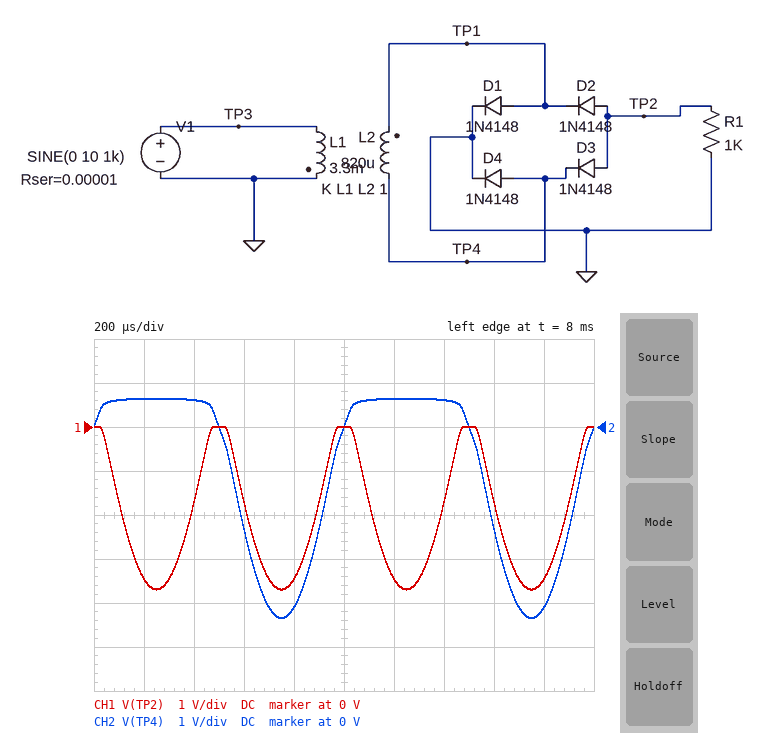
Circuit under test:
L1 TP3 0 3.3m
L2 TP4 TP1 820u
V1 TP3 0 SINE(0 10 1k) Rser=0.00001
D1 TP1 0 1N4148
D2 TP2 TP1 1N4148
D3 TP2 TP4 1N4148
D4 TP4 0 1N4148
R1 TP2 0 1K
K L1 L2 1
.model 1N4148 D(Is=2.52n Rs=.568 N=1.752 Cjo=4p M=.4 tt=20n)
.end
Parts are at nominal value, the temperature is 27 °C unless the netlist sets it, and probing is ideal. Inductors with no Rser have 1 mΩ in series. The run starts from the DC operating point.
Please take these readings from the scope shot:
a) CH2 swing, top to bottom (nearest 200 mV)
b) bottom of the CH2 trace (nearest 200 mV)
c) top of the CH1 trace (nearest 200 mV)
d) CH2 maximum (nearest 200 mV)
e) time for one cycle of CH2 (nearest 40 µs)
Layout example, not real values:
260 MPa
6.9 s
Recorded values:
5.0 V
-4.4 V
0 V
600 mV
1.00 ms
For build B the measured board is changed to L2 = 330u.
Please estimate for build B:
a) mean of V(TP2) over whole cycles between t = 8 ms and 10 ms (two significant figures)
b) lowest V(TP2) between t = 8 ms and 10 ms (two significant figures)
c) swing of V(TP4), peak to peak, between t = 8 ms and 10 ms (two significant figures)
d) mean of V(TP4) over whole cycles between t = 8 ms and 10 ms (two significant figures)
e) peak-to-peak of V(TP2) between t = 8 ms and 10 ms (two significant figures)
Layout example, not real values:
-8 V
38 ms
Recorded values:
-980 mV
-1.9 V
3.2 V
-490 mV
1.9 V
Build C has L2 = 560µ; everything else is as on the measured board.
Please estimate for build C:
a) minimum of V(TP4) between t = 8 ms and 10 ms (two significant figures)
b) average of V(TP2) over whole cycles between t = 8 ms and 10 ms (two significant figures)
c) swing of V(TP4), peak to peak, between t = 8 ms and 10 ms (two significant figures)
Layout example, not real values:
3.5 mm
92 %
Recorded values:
-3.5 V
-1.5 V
4.1 V
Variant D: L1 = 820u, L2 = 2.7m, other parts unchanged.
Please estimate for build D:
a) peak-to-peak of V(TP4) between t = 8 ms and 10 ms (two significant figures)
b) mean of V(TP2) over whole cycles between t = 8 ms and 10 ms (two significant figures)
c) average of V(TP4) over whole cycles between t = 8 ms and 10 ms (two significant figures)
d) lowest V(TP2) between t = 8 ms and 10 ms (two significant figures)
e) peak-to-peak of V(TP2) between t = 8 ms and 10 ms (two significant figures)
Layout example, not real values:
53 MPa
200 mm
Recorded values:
18 V
-10 V
-5.1 V
-17 V
17 V
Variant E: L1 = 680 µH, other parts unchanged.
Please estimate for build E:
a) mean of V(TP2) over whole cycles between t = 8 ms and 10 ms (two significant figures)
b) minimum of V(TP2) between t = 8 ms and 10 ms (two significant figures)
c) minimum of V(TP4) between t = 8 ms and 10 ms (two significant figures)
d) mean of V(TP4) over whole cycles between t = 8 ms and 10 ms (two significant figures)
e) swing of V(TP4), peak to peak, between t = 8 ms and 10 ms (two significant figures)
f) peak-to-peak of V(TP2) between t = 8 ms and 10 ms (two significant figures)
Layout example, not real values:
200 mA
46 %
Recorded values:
-5.7 V
-9.6 V
-10 V
-2.9 V
11 V
9.6 V
